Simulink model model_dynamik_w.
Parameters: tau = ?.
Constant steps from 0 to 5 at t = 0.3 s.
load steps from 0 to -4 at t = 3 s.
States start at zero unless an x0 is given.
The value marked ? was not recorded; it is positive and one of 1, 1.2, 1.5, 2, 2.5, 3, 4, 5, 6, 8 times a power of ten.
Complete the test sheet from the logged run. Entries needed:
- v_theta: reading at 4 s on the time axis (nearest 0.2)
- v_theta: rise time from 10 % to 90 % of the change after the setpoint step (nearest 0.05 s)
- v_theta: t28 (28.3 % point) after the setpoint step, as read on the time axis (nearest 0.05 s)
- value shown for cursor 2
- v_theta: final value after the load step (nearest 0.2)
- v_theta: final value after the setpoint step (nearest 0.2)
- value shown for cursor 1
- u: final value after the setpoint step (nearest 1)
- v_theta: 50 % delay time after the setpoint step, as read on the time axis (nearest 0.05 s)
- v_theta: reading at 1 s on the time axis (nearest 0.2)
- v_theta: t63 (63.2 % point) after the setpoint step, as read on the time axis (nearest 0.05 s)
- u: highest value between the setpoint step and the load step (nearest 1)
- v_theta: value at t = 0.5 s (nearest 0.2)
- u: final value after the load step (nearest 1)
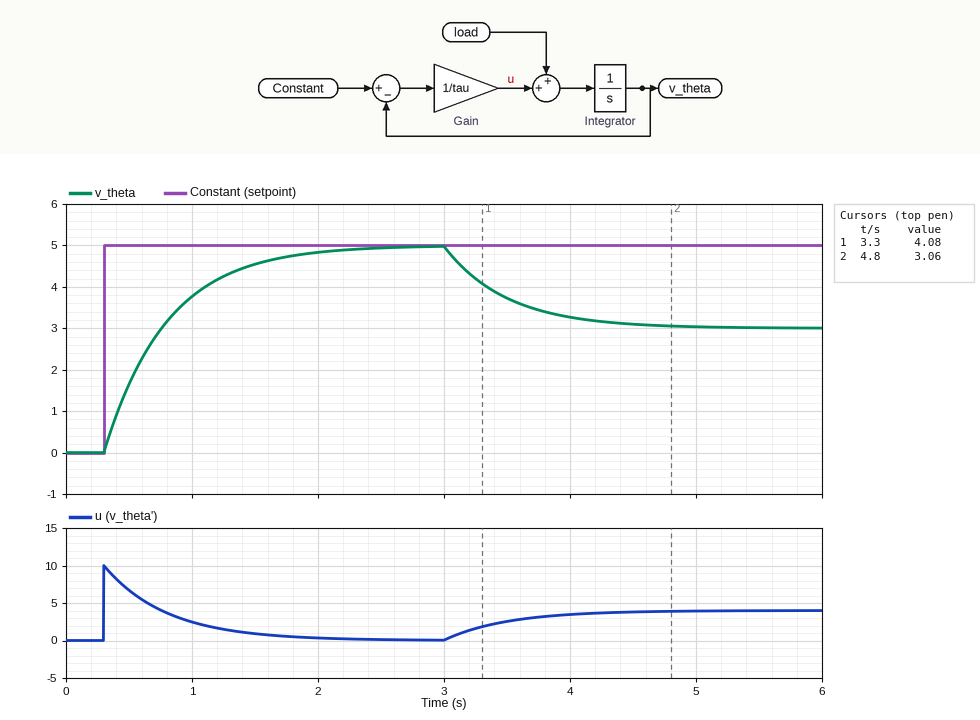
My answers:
3.2
1.10 s
0.45 s
3.06
3.0
5.0
4.08
0
0.65 s
3.8
0.80 s
10
1.6
4
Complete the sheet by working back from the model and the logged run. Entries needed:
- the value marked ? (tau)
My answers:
0.5
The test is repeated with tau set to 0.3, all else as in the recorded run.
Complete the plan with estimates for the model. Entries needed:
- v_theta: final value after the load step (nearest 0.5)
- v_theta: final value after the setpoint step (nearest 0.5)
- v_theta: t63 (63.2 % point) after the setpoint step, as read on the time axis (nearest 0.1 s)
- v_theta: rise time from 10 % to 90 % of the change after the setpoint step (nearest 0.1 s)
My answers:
4.0
5.0
0.6 s
0.7 s
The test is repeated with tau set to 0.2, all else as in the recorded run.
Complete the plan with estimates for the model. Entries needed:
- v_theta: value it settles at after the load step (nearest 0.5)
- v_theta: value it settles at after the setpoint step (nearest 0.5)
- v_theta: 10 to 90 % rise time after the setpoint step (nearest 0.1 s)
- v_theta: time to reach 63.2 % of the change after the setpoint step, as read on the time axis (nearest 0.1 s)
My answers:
4.0
5.0
0.4 s
0.5 s
